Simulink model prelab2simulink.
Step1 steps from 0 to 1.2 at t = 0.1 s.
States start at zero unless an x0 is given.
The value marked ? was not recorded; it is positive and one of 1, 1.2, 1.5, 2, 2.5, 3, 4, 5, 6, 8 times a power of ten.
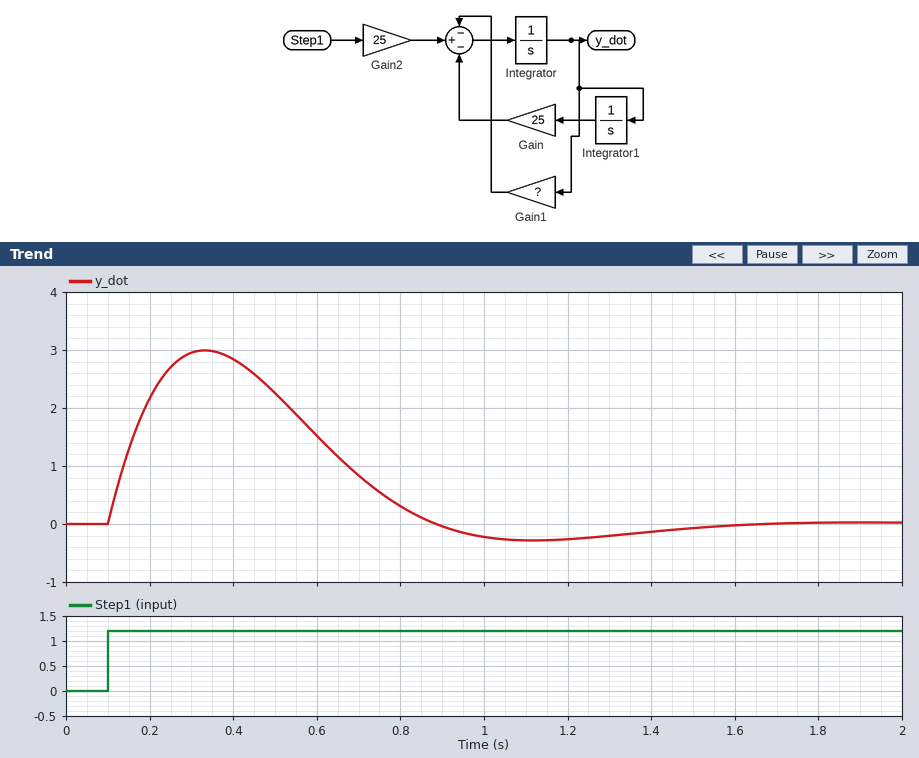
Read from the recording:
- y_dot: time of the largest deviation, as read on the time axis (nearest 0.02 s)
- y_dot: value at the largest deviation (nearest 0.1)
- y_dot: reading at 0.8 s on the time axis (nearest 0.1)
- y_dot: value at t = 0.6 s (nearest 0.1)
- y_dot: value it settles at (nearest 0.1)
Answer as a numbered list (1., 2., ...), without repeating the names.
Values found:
1. 0.34 s
2. 3.0
3. 0.3
4. 1.5
5. 0.0
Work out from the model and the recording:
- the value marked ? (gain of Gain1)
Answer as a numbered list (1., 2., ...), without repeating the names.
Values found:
1. 6
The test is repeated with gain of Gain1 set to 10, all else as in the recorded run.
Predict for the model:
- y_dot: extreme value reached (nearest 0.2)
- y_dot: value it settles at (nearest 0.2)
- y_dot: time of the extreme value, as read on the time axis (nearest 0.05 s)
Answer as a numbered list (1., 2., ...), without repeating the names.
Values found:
1. 2.2
2. 0.0
3. 0.30 s
